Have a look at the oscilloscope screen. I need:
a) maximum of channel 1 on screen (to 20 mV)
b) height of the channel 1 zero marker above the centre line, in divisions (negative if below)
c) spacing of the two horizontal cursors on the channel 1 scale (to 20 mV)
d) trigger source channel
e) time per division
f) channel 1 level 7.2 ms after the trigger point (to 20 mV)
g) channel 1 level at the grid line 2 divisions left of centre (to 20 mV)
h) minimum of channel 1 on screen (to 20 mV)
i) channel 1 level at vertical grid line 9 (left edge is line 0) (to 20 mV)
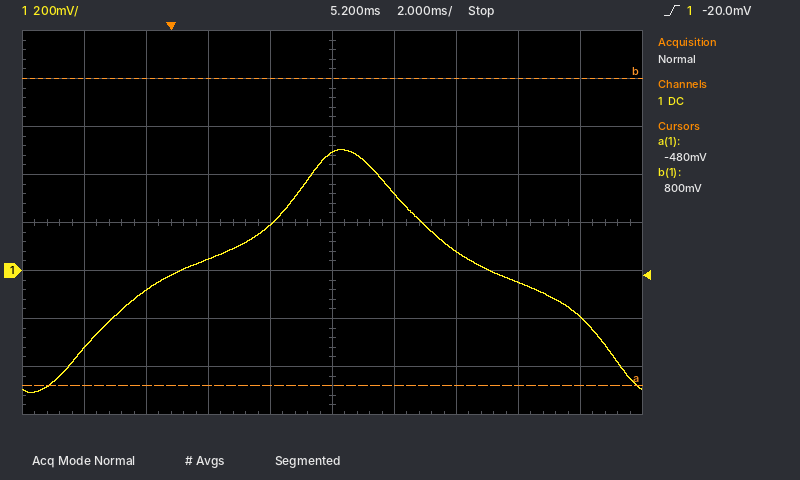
500 mV
-1.0 div
1.28 V
channel 1
2 ms
320 mV
40 mV
-500 mV
-200 mV
